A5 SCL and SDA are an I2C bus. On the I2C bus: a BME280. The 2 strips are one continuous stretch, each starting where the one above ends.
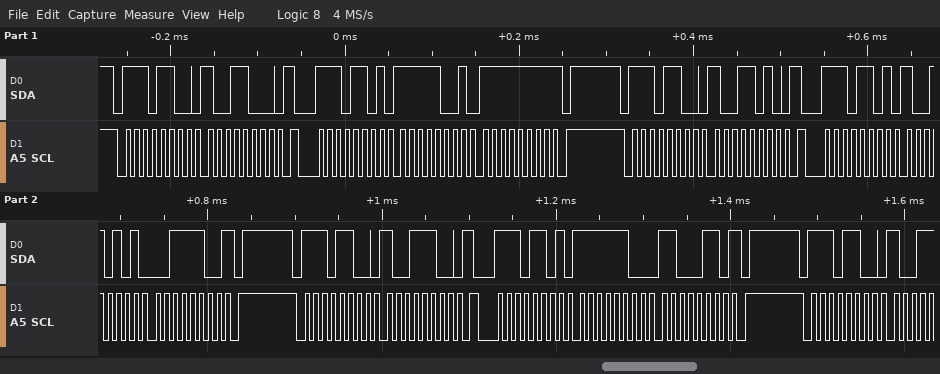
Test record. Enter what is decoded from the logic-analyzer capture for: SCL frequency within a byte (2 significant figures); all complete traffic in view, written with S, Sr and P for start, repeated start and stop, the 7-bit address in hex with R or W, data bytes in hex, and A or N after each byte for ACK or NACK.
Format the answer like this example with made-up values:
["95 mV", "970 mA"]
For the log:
["100 kHz", "S 76W A 98 A Sr 76R A F9 A FF N P S 76W A 9A A Sr 76R A 95 A 3C N P S 76W A 9C A Sr 76R A FC A C6 N P S 76W A"]
